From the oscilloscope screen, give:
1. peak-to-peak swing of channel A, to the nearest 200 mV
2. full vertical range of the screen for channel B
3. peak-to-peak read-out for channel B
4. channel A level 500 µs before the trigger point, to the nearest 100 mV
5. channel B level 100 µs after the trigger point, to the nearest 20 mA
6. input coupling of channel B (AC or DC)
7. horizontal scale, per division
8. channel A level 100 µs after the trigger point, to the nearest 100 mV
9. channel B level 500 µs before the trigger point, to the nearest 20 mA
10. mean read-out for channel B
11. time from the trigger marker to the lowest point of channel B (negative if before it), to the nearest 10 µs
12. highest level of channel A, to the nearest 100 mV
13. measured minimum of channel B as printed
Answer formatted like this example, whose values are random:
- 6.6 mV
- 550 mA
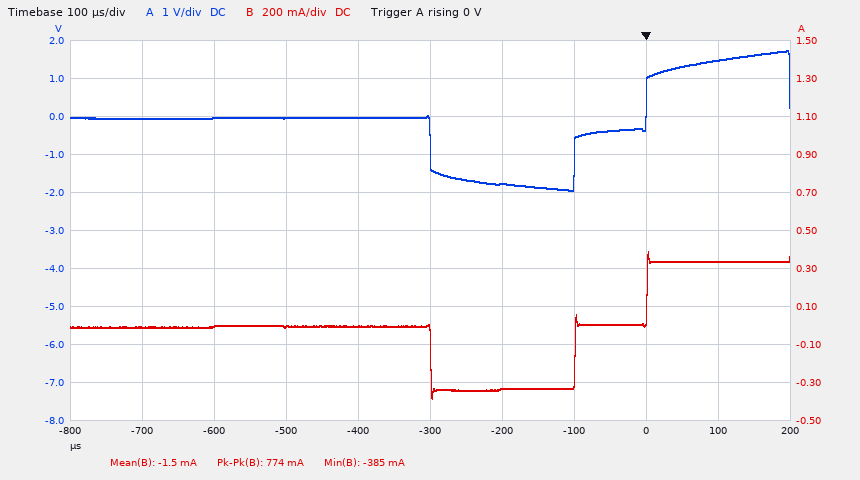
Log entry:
- 3.6 V
- 2 A
- 774 mA
- 0.0 V
- 340 mA
- DC
- 100 µs
- 1.5 V
- 0 mA
- -1.5 mA
- -300 µs
- 1.7 V
- -385 mA
